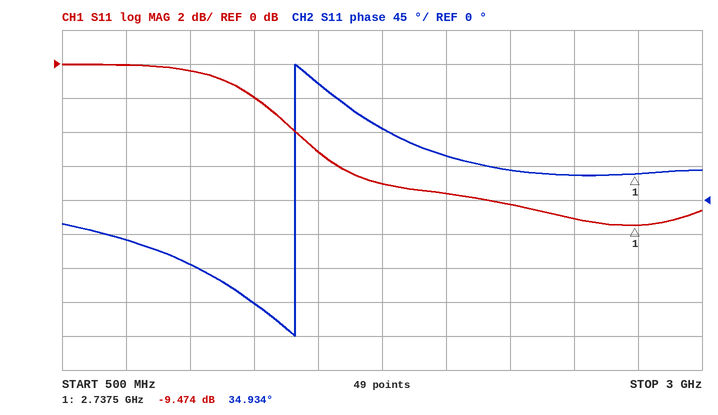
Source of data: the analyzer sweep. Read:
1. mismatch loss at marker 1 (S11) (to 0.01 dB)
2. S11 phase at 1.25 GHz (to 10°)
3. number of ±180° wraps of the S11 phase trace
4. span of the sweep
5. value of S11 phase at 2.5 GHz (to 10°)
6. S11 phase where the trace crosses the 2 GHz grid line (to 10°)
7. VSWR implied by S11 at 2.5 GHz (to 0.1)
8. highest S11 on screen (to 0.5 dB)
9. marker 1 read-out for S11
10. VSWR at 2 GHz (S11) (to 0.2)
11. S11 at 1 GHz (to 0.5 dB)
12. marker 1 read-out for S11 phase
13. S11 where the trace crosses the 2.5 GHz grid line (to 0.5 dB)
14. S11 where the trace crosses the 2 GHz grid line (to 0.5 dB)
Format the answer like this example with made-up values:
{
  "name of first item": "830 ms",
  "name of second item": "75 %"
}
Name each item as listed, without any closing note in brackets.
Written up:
{
  "mismatch loss at marker 1 (S11)": "0.52 dB",
  "S11 phase at 1.25 GHz": "-140°",
  "number of ±180° wraps of the S11 phase trace": "1",
  "span of the sweep": "2.5 GHz",
  "value of S11 phase at 2.5 GHz": "30°",
  "S11 phase where the trace crosses the 2 GHz grid line": "60°",
  "VSWR implied by S11 at 2.5 GHz": "2.1",
  "highest S11 on screen": "0.0 dB",
  "marker 1 read-out for S11": "-9.474 dB",
  "VSWR at 2 GHz (S11)": "2.4",
  "S11 at 1 GHz": "-0.5 dB",
  "marker 1 read-out for S11 phase": "34.934°",
  "S11 where the trace crosses the 2.5 GHz grid line": "-9.0 dB",
  "S11 where the trace crosses the 2 GHz grid line": "-7.5 dB"
}
